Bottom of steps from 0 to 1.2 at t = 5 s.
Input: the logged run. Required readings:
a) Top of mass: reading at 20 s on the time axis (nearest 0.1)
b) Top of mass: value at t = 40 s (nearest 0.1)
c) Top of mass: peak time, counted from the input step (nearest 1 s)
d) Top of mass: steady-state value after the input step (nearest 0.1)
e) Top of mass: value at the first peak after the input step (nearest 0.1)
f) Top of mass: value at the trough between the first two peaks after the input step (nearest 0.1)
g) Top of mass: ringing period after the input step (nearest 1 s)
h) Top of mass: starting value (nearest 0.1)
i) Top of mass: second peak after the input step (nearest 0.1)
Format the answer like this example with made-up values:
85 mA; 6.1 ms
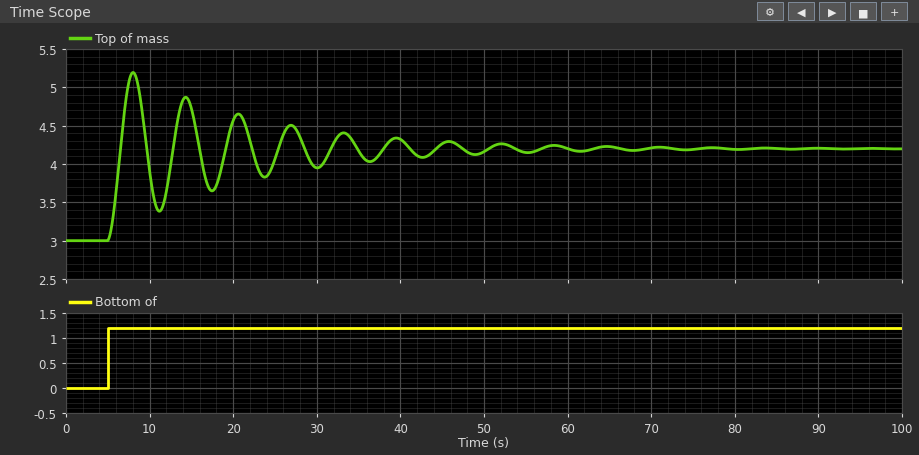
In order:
4.6; 4.3; 3 s; 4.2; 5.2; 3.4; 6 s; 3.0; 4.9
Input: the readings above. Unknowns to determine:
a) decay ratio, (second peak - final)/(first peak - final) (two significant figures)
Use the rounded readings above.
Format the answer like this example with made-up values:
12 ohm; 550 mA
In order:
0.70
